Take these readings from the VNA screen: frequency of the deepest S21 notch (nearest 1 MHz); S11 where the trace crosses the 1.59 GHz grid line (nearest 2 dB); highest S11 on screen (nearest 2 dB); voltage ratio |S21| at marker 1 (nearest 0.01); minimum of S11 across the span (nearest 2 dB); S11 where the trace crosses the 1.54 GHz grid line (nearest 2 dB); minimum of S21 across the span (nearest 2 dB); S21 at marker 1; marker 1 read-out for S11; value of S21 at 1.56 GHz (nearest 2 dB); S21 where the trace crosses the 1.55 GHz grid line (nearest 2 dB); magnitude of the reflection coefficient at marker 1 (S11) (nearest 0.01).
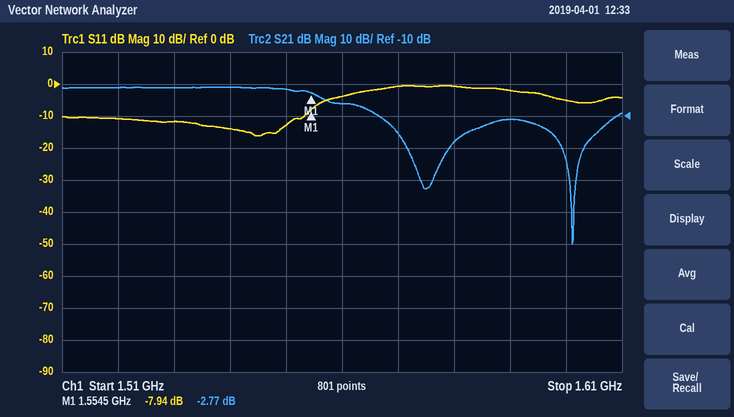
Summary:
1.601 GHz
-2 dB
0 dB
0.73
-16 dB
-14 dB
-50 dB
-2.77 dB
-7.94 dB
-6 dB
-2 dB
0.40
